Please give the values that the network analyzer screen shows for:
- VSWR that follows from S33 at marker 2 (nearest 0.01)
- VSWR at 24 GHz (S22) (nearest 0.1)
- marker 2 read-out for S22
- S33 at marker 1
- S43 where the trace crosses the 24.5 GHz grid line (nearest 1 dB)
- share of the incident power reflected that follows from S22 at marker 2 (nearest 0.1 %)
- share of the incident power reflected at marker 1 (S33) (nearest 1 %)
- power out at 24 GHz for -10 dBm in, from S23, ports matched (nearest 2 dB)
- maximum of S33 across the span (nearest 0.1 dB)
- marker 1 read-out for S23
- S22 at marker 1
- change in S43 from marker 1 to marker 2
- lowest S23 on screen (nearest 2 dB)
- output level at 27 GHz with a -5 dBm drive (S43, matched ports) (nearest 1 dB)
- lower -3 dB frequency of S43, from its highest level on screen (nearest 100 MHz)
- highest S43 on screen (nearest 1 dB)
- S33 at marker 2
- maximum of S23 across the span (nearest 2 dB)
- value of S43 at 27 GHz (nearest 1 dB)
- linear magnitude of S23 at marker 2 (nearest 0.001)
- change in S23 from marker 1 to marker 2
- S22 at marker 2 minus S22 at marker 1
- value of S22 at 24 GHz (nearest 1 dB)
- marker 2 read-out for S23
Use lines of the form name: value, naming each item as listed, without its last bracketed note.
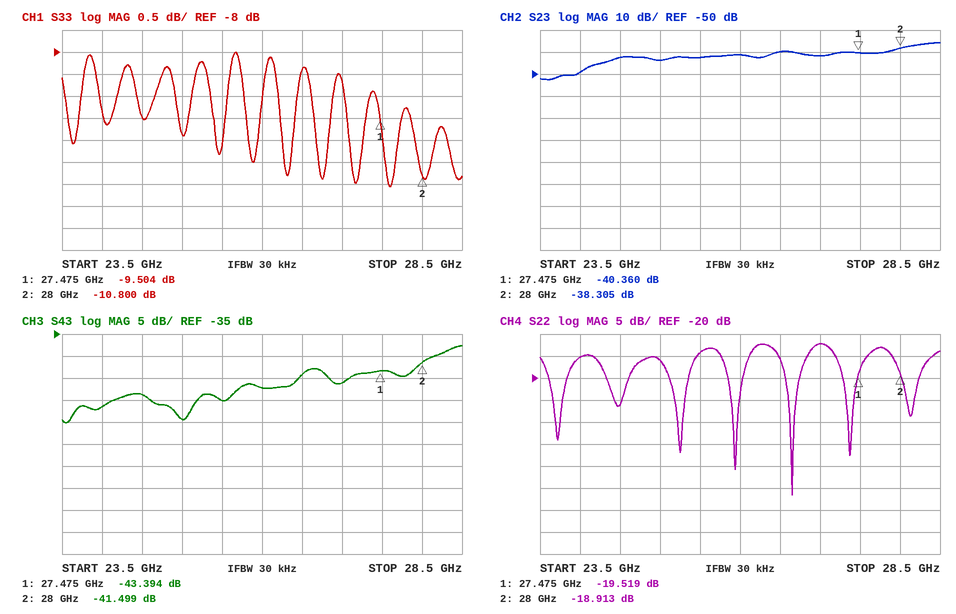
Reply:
VSWR that follows from S33 at marker 2: 1.81
VSWR at 24 GHz (S22): 1.4
marker 2 read-out for S22: -18.913 dB
S33 at marker 1: -9.504 dB
S43 where the trace crosses the 24.5 GHz grid line: -49 dB
share of the incident power reflected that follows from S22 at marker 2: 1.3 %
share of the incident power reflected at marker 1 (S33): 11 %
power out at 24 GHz for -10 dBm in, from S23, ports matched: -60 dBm
maximum of S33 across the span: -8.0 dB
marker 1 read-out for S23: -40.360 dB
S22 at marker 1: -19.519 dB
change in S43 from marker 1 to marker 2: 1.895 dB
lowest S23 on screen: -52 dB
output level at 27 GHz with a -5 dBm drive (S43, matched ports): -51 dBm
lower -3 dB frequency of S43, from its highest level on screen: 28.1 GHz
highest S43 on screen: -38 dB
S33 at marker 2: -10.800 dB
maximum of S23 across the span: -36 dB
value of S43 at 27 GHz: -46 dB
linear magnitude of S23 at marker 2: 0.012
change in S23 from marker 1 to marker 2: 2.055 dB
S22 at marker 2 minus S22 at marker 1: 0.606 dB
value of S22 at 24 GHz: -15 dB
marker 2 read-out for S23: -38.305 dB
